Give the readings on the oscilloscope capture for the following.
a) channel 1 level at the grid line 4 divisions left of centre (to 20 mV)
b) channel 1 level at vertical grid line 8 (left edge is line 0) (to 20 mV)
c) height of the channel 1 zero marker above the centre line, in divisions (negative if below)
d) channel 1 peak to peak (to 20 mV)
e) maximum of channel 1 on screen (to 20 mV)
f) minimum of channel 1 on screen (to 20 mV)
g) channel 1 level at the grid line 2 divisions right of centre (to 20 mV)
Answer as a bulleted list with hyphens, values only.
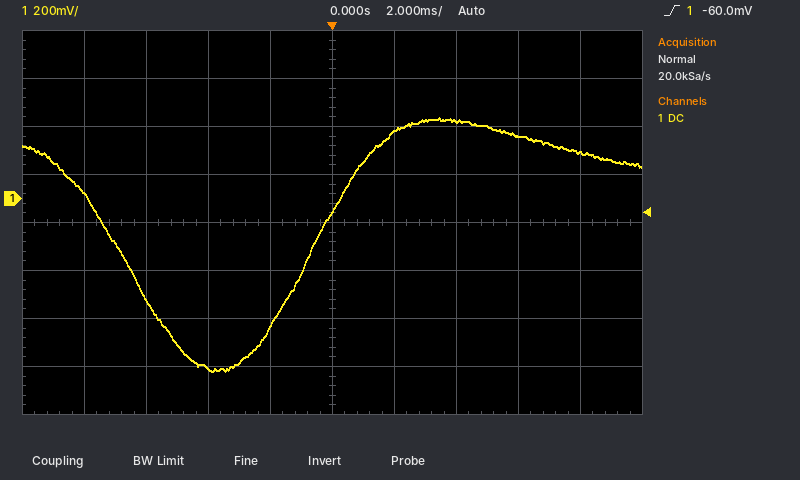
- 20 mV
- 260 mV
- +0.5 div
- 1.06 V
- 340 mV
- -720 mV
- 320 mV
